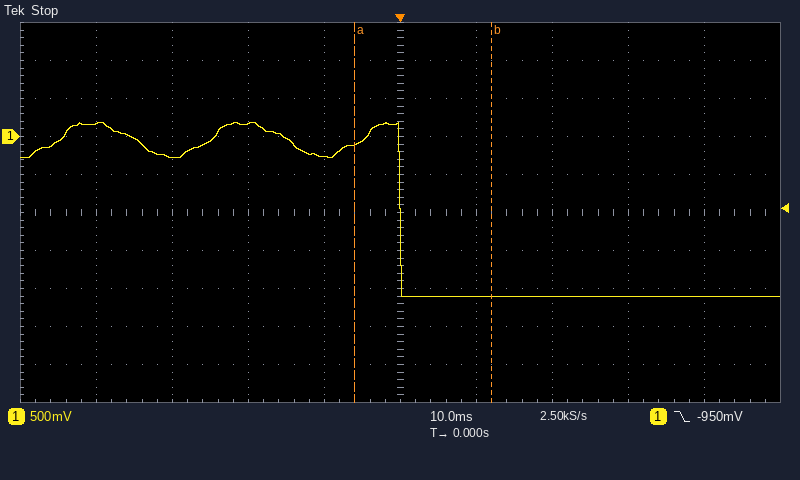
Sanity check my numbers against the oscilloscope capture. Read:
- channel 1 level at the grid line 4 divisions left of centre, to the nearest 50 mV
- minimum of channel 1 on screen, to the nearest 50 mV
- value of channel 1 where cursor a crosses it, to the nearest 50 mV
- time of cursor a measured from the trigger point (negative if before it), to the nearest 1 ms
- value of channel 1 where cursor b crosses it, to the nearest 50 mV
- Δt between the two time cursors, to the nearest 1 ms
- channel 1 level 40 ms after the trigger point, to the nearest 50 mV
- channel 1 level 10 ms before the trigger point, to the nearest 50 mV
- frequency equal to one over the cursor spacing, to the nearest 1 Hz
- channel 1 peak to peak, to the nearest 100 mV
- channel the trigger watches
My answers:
150 mV
-2.10 V
-100 mV
-6 ms
-2.10 V
18 ms
-2.10 V
-250 mV
56 Hz
2.30 V
channel 1
